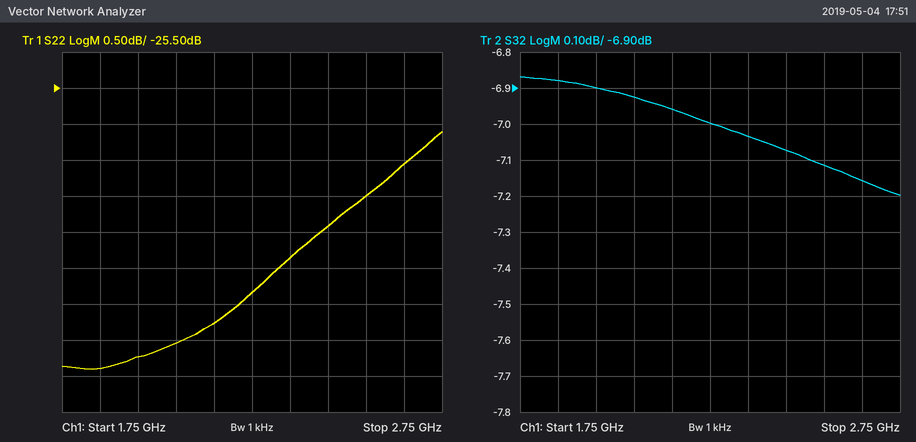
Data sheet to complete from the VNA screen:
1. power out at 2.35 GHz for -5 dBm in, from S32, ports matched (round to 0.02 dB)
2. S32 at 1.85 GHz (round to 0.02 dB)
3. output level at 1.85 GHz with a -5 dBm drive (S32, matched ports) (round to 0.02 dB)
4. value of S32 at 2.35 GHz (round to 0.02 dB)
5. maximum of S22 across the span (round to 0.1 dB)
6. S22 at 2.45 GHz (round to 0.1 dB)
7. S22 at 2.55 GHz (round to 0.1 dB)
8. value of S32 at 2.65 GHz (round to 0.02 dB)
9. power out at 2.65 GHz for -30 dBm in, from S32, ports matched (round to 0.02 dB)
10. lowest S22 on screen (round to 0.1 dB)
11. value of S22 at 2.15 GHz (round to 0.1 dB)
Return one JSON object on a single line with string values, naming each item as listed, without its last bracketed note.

{"power out at 2.35 GHz for -5 dBm in, from S32, ports matched": "-12.04 dBm", "S32 at 1.85 GHz": "-6.88 dB", "output level at 1.85 GHz with a -5 dBm drive (S32, matched ports)": "-11.88 dBm", "value of S32 at 2.35 GHz": "-7.04 dB", "maximum of S22 across the span": "-26.1 dB", "S22 at 2.45 GHz": "-27.4 dB", "S22 at 2.55 GHz": "-27.0 dB", "value of S32 at 2.65 GHz": "-7.16 dB", "power out at 2.65 GHz for -30 dBm in, from S32, ports matched": "-37.16 dBm", "lowest S22 on screen": "-29.4 dB", "value of S22 at 2.15 GHz": "-28.8 dB"}
